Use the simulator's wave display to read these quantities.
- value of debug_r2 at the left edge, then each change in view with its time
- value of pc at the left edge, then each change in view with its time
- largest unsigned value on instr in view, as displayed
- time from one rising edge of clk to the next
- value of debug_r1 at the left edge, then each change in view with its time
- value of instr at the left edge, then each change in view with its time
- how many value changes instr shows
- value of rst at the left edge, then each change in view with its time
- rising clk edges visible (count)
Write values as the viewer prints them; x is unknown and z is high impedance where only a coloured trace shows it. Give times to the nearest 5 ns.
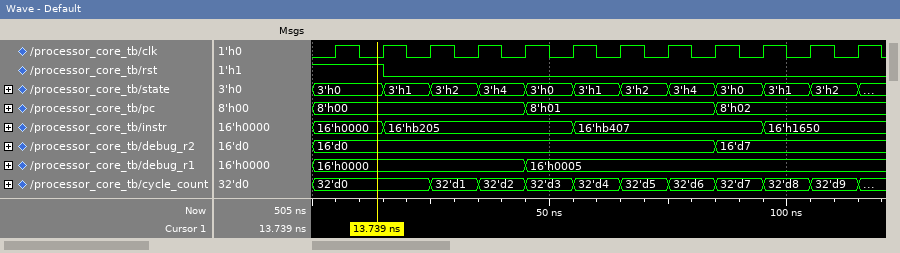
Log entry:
16'd0, 16'd7 at 85 ns
8'h00, 8'h01 at 45 ns, 8'h02 at 85 ns
16'hb407
10 ns
16'h0000, 16'h0005 at 45 ns
16'h0000, 16'hb205 at 15 ns, 16'hb407 at 55 ns, 16'h1650 at 95 ns
3
1, 0 at 15 ns
12
